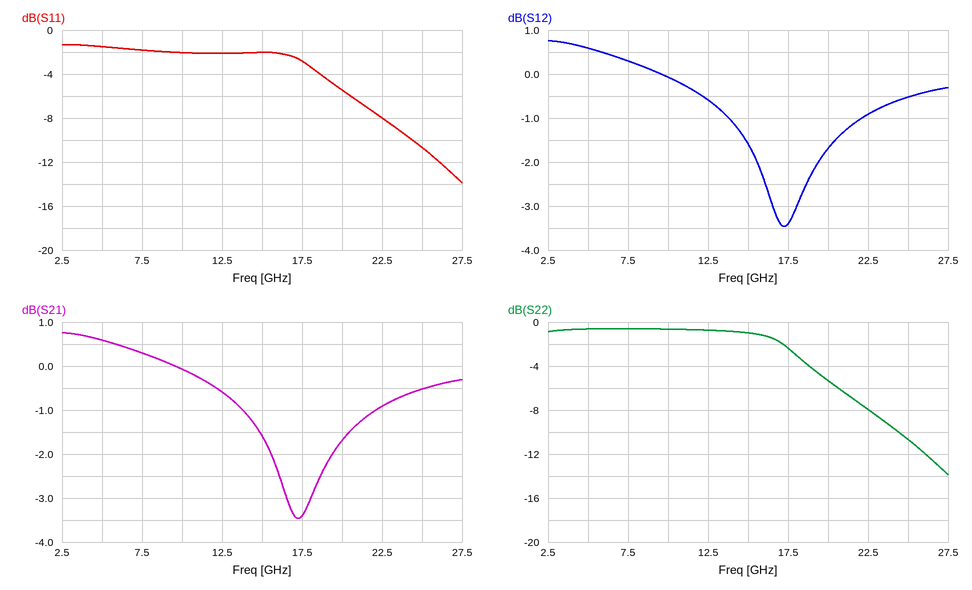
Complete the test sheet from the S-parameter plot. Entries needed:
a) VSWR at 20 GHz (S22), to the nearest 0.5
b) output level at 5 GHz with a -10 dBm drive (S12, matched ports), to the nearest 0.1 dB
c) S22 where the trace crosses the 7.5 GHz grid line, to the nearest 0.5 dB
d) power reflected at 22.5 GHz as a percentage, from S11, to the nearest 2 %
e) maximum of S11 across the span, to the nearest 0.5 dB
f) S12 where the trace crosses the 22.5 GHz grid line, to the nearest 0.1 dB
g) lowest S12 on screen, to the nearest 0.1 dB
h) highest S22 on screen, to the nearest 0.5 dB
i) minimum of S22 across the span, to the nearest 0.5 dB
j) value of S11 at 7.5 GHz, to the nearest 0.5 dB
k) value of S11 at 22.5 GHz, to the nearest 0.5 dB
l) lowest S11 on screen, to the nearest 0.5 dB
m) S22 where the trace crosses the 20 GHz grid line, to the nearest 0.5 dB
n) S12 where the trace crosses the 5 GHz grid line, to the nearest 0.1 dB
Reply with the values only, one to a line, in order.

3.5
-9.4 dBm
-0.5 dB
16 %
-1.5 dB
-0.9 dB
-3.5 dB
-0.5 dB
-14.0 dB
-2.0 dB
-8.0 dB
-14.0 dB
-5.5 dB
0.6 dB
